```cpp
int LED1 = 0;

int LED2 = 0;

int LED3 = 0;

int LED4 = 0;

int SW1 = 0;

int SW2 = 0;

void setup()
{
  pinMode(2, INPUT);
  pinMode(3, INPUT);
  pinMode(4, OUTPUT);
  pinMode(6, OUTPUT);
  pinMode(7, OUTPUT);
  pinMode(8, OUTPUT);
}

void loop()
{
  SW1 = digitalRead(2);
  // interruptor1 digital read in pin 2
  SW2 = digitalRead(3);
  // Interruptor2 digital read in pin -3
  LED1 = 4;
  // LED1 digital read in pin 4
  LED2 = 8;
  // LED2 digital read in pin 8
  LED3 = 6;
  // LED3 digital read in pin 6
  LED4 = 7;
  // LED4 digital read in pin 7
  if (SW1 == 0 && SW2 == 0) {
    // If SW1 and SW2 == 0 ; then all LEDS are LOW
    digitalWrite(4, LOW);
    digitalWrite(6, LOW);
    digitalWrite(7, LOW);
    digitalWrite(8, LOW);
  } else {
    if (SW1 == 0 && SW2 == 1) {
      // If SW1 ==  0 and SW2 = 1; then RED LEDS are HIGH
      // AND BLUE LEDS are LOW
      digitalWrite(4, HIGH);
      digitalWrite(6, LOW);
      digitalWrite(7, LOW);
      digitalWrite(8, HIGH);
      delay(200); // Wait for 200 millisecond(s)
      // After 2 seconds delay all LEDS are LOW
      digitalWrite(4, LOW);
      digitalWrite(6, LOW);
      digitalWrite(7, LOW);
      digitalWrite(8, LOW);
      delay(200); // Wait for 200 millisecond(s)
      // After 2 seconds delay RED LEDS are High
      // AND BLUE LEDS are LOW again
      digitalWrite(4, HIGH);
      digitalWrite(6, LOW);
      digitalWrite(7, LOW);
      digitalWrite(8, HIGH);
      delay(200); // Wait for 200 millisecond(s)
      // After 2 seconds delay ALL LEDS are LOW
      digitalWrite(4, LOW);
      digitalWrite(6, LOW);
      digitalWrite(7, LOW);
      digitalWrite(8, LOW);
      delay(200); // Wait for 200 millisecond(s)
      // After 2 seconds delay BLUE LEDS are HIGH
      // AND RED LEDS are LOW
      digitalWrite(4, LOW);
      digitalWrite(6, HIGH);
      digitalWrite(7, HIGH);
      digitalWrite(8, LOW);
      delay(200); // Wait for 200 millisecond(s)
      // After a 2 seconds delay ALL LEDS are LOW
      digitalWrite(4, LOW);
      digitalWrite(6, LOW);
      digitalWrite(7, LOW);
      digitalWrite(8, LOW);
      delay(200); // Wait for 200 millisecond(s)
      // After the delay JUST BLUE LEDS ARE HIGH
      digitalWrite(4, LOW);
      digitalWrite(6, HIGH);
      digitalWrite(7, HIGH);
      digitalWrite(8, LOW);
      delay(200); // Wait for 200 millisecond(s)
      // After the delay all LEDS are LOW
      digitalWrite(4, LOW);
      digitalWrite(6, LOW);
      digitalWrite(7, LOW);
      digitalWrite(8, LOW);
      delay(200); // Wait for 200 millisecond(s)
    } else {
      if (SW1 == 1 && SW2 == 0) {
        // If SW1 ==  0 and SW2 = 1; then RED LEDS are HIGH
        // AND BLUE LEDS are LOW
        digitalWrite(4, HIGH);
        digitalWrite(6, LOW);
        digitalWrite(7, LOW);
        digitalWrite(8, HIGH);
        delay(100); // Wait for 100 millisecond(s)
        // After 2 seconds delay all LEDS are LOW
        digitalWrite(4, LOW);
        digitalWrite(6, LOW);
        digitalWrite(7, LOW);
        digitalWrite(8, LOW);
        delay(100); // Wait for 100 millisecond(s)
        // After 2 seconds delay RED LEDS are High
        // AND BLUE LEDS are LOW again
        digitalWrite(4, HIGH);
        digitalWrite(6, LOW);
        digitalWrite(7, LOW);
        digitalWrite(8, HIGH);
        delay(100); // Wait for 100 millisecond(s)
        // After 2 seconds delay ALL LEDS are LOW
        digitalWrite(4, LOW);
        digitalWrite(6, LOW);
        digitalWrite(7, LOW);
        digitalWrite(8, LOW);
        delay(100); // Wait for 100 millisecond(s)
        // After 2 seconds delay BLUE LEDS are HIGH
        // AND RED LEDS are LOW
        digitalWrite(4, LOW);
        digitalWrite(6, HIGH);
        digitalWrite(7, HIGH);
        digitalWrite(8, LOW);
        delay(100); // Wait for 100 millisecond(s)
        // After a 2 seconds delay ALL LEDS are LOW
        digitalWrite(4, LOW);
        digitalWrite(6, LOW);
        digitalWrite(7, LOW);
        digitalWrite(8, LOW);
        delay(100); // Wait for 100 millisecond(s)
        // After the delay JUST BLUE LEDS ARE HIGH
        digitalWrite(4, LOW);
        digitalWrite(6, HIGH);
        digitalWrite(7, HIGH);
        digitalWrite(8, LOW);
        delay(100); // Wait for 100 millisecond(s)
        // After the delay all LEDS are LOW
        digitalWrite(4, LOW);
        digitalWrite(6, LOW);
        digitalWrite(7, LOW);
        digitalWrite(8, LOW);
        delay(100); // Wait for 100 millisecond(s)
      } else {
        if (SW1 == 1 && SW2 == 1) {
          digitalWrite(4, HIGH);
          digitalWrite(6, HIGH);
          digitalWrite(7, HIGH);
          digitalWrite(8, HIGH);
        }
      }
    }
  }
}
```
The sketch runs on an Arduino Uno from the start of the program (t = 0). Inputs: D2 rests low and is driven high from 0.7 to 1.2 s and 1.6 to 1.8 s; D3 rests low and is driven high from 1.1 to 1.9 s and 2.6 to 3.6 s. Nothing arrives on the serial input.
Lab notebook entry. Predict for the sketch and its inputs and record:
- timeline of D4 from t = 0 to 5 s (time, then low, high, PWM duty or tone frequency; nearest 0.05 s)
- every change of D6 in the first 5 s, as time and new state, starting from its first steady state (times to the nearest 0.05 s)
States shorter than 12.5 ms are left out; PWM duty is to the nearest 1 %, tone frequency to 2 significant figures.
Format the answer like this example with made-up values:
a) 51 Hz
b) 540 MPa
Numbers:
a) 0 s low; 0.7 s high; 0.8 s low; 0.9 s high; 1 s low; 1.5 s high; 1.7 s low; 1.9 s high; 2.1 s low; 3.1 s high; 3.3 s low; 3.5 s high; 3.7 s low
b) 0 s low; 1.1 s high; 1.2 s low; 1.3 s high; 1.4 s low; 2.3 s high; 2.5 s low; 2.7 s high; 2.9 s low; 3.9 s high; 4.1 s low; 4.3 s high; 4.5 s low
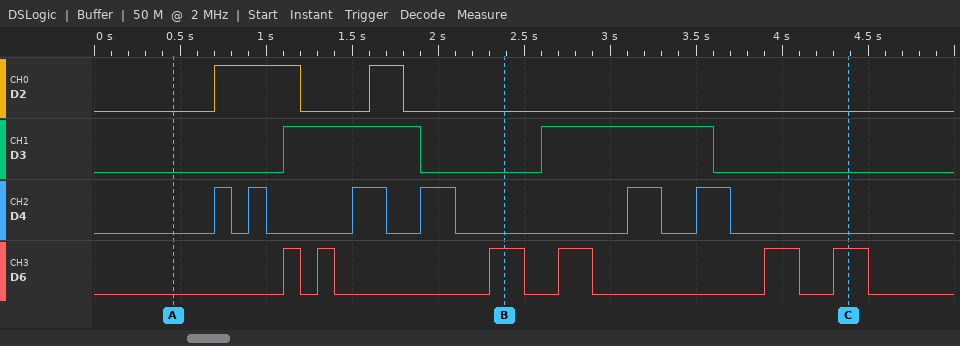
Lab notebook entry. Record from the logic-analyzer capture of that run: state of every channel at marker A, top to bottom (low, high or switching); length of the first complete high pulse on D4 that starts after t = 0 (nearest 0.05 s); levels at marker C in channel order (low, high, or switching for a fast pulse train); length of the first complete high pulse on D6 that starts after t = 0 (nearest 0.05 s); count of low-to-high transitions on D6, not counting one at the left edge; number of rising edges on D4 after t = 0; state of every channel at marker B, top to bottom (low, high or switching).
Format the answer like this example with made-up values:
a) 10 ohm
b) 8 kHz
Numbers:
a) D2 low, D3 low, D4 low, D6 low
b) 0.10 s
c) D2 low, D3 low, D4 low, D6 high
d) 0.10 s
e) 6
f) 6
g) D2 low, D3 low, D4 low, D6 high
